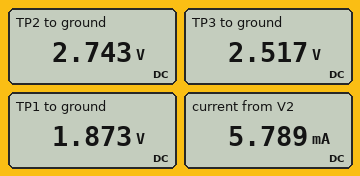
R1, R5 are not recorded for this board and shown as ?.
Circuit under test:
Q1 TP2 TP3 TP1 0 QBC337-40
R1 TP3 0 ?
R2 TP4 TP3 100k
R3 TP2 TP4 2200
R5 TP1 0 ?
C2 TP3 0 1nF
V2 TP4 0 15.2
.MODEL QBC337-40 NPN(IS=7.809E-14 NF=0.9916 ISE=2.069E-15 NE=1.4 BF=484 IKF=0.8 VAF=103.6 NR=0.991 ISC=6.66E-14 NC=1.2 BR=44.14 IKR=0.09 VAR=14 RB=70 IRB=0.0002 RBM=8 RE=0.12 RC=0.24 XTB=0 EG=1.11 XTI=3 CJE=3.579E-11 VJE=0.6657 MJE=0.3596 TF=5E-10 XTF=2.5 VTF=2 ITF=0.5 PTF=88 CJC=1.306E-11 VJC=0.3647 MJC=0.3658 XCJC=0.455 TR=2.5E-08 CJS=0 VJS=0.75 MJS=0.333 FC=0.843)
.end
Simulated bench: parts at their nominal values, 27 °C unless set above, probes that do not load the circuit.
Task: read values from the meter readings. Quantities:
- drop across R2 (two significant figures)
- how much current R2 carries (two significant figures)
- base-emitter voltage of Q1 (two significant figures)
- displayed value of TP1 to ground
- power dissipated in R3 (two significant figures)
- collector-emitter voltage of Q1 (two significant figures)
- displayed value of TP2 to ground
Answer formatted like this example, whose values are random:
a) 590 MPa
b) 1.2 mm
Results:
a) 13 V
b) 130 µA
c) 640 mV
d) 1.873 V
e) 71 mW
f) 870 mV
g) 2.743 V
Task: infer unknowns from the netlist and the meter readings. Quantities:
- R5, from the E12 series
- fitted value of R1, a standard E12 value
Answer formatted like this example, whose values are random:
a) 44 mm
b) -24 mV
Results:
a) 330 Ω
b) 22 kΩ
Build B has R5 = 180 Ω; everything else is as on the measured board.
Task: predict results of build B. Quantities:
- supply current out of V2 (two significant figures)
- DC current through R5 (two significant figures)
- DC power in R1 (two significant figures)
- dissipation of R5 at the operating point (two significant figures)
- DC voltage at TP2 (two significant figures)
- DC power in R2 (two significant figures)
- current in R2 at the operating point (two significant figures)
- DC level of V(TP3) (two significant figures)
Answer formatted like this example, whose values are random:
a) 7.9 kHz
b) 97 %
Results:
a) 6.5 mA
b) 6.4 mA
c) 150 µW
d) 7.4 mW
e) 1.2 V
f) 1.8 mW
g) 130 µA
h) 1.8 V
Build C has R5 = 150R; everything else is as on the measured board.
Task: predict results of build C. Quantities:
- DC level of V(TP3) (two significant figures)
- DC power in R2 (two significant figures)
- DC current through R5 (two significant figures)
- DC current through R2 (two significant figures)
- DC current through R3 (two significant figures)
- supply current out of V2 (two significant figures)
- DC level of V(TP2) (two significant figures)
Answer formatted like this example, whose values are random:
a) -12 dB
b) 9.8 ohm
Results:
a) 1.6 V
b) 1.8 mW
c) 6.5 mA
d) 140 µA
e) 6.4 mA
f) 6.6 mA
g) 1.0 V
